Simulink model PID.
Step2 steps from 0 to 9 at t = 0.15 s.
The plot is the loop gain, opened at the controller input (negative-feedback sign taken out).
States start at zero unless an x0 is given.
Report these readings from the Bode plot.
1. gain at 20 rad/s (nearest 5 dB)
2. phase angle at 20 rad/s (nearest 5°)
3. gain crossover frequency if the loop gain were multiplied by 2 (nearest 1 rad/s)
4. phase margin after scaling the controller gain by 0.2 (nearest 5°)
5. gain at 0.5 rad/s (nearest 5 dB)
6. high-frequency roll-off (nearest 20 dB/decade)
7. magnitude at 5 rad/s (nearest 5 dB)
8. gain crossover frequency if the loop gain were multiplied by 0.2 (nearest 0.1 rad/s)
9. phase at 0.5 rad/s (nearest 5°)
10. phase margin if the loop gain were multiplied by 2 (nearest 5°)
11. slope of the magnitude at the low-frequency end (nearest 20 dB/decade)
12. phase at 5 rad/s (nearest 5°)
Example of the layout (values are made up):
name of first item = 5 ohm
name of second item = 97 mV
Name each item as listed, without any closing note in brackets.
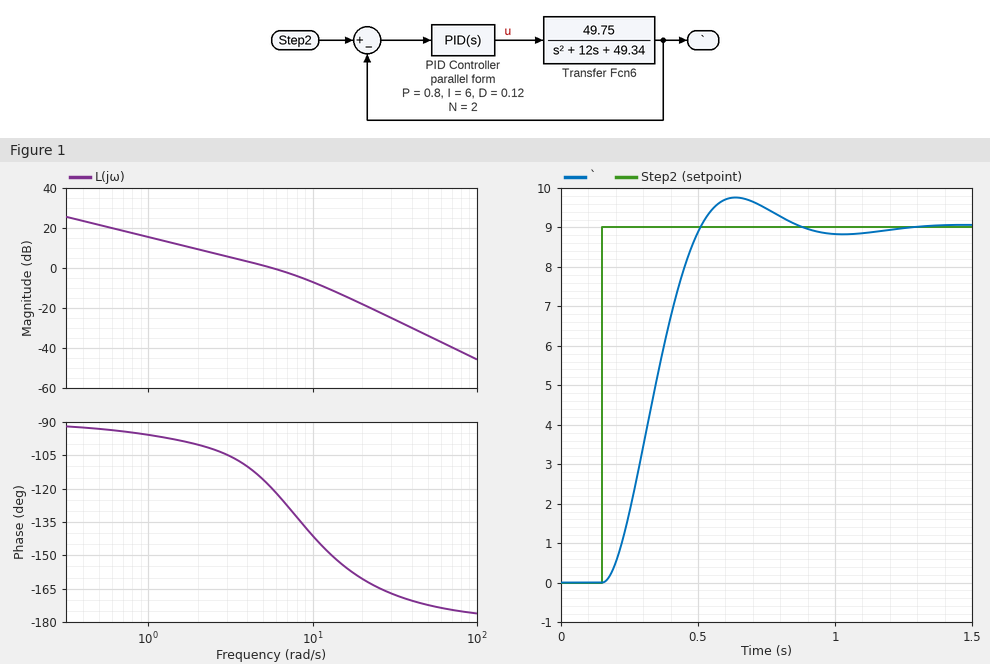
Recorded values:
gain at 20 rad/s = -20 dB
phase angle at 20 rad/s = -160°
gain crossover frequency if the loop gain were multiplied by 2 = 9 rad/s
phase margin after scaling the controller gain by 0.2 = 85°
gain at 0.5 rad/s = 20 dB
high-frequency roll-off = -40 dB/decade
magnitude at 5 rad/s = 0 dB
gain crossover frequency if the loop gain were multiplied by 0.2 = 1.2 rad/s
phase at 0.5 rad/s = -95°
phase margin if the loop gain were multiplied by 2 = 40°
slope of the magnitude at the low-frequency end = -20 dB/decade
phase at 5 rad/s = -115°
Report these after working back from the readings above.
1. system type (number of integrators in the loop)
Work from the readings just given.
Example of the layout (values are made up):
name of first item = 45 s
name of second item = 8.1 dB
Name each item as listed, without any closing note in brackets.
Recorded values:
system type = 1
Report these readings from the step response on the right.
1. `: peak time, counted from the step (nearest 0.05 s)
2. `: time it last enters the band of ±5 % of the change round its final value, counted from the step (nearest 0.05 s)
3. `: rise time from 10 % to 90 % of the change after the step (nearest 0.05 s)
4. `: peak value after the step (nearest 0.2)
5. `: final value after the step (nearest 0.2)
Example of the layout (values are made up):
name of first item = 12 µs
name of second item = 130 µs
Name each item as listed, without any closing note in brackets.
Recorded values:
`: peak time, counted from the step = 0.50 s
`: time it last enters the band of ±5 % of the change round its final value, counted from the step = 0.60 s
`: rise time from 10 % to 90 % of the change after the step = 0.25 s
`: peak value after the step = 9.8
`: final value after the step = 9.0
